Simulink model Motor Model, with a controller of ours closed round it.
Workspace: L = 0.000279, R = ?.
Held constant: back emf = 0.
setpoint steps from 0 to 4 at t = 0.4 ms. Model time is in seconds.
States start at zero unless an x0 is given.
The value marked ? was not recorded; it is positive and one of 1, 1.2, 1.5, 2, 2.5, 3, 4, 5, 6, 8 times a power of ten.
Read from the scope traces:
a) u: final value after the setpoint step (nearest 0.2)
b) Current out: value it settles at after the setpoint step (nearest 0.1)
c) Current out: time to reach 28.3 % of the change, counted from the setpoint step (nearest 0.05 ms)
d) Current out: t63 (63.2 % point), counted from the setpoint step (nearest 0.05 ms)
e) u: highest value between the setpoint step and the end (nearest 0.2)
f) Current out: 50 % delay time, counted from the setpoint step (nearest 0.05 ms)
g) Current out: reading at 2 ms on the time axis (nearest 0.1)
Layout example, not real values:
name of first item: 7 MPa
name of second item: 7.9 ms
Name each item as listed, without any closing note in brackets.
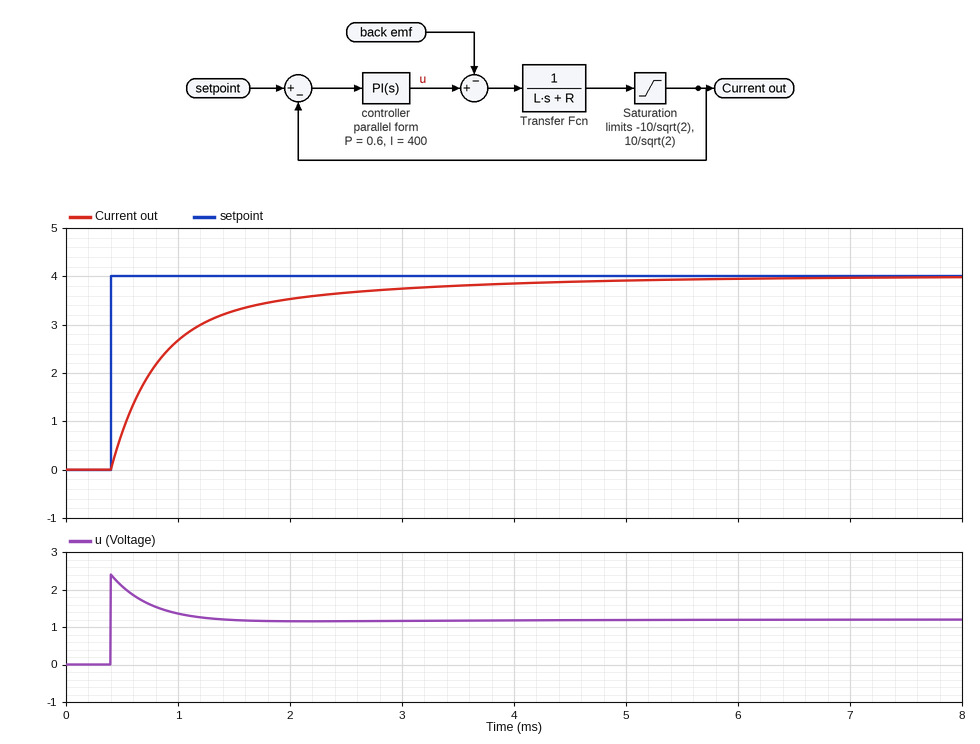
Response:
u: final value after the setpoint step: 1.2
Current out: value it settles at after the setpoint step: 4.0
Current out: time to reach 28.3 % of the change, counted from the setpoint step: 0.15 ms
Current out: t63 (63.2 % point), counted from the setpoint step: 0.55 ms
u: highest value between the setpoint step and the end: 2.4
Current out: 50 % delay time, counted from the setpoint step: 0.35 ms
Current out: reading at 2 ms on the time axis: 3.5
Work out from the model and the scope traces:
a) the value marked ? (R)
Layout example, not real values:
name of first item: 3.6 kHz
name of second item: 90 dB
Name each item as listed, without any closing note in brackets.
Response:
the value marked ?: 0.3
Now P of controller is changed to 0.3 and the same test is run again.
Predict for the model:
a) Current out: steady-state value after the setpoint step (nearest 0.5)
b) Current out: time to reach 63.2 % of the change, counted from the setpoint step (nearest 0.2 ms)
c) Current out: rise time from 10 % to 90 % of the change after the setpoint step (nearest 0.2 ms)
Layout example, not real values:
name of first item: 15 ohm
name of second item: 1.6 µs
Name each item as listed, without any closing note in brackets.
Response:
Current out: steady-state value after the setpoint step: 4.0
Current out: time to reach 63.2 % of the change, counted from the setpoint step: 0.8 ms
Current out: rise time from 10 % to 90 % of the change after the setpoint step: 1.6 ms
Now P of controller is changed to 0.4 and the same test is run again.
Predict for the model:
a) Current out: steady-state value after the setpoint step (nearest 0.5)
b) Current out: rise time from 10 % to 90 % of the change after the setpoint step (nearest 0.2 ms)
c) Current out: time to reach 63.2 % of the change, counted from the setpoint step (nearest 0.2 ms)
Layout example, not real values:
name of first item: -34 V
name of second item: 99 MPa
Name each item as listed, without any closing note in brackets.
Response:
Current out: steady-state value after the setpoint step: 4.0
Current out: rise time from 10 % to 90 % of the change after the setpoint step: 1.6 ms
Current out: time to reach 63.2 % of the change, counted from the setpoint step: 0.8 ms
